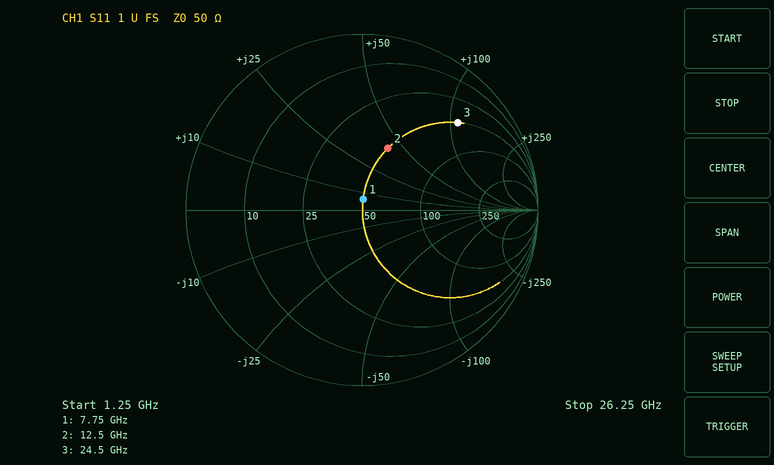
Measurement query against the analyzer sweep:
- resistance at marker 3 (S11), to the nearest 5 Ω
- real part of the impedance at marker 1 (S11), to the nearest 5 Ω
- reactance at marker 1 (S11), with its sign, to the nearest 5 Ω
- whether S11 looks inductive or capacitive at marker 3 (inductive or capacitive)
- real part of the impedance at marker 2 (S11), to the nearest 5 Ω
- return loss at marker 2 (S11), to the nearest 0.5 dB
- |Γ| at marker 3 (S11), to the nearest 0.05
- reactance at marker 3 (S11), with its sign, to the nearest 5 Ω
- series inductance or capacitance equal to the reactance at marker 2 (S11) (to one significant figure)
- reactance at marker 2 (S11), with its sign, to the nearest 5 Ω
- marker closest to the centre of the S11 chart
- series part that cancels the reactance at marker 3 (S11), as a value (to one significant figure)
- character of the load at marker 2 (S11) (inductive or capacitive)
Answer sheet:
50 Ω
50 Ω
+5 Ω
inductive
50 Ω
8.5 dB
0.75
+110 Ω
500 pH
+40 Ω
marker 1
60 fF
inductive
